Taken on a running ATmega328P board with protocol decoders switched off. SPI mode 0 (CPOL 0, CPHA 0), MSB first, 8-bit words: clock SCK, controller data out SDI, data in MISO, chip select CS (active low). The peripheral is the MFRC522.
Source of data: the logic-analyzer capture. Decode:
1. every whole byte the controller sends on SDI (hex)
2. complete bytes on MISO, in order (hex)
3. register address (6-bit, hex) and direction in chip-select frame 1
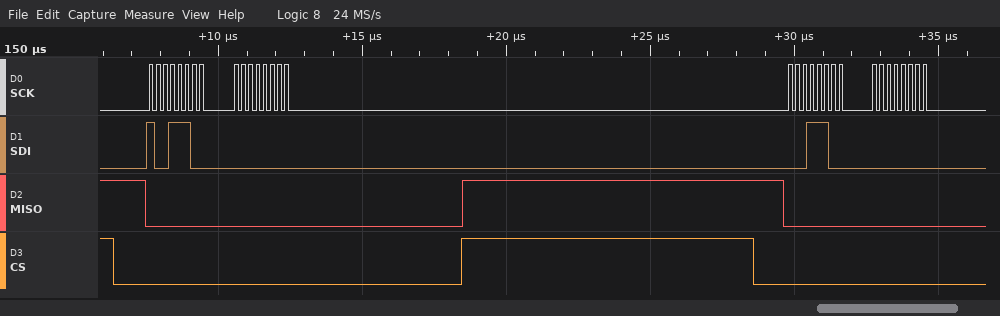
0x9C 0x00 0x1C 0x00
0x00 0x00 0x00 0x00
0x0E read
